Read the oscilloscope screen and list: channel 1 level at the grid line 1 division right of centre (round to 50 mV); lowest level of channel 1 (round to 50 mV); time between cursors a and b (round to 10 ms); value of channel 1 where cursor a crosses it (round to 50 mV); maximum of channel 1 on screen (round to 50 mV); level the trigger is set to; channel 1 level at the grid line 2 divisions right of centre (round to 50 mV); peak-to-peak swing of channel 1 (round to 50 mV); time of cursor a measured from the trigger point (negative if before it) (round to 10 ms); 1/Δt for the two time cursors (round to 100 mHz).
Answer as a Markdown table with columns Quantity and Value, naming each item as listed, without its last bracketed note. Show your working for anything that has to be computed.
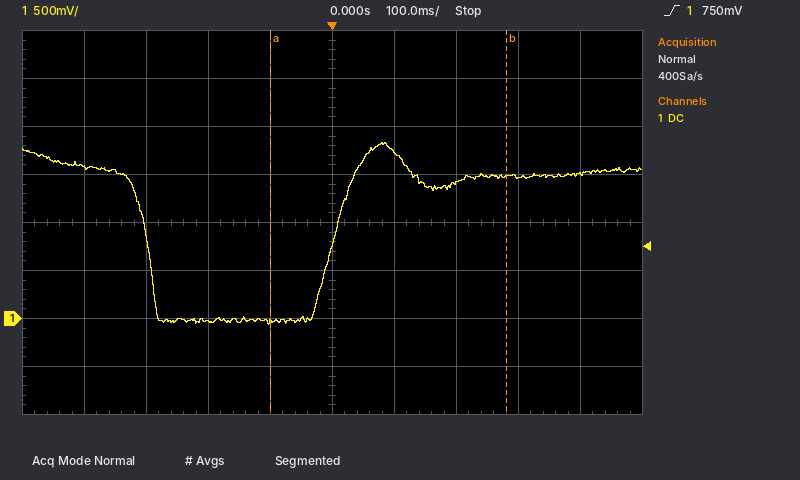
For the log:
| Quantity | Value |
|---|---|
| channel 1 level at the grid line 1 division right of centre | 1.75 V |
| lowest level of channel 1 | -50 mV |
| time between cursors a and b | 380 ms |
| value of channel 1 where cursor a crosses it | -50 mV |
| maximum of channel 1 on screen | 1.85 V |
| level the trigger is set to | 750 mV |
| channel 1 level at the grid line 2 divisions right of centre | 1.40 V |
| peak-to-peak swing of channel 1 | 1.85 V − (-50 mV) = 1.90 V |
| time of cursor a measured from the trigger point (negative if before it) | -100 ms |
| 1/Δt for the two time cursors | 1 / 380 ms ≈ 2.6 Hz |
